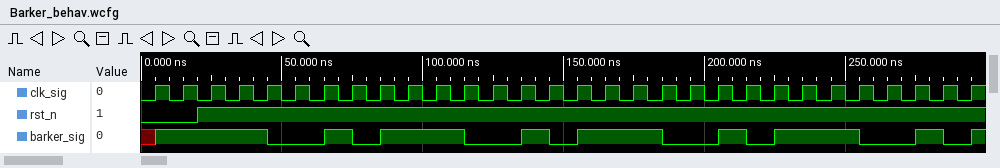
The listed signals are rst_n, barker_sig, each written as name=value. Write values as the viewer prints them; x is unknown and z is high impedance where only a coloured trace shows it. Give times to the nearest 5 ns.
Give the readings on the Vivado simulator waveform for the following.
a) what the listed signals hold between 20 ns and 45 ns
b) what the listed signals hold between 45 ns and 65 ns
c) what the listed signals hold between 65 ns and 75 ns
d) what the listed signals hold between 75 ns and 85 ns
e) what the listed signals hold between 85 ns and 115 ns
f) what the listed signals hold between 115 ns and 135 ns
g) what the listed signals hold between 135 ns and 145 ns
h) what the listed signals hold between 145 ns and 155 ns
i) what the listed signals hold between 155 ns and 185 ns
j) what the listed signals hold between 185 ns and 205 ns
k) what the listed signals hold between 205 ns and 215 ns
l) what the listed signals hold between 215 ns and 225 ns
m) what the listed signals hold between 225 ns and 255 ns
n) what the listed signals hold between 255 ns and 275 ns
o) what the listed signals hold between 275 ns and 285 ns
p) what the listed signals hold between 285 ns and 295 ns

rst_n=1, barker_sig=1
rst_n=1, barker_sig=0
rst_n=1, barker_sig=1
rst_n=1, barker_sig=0
rst_n=1, barker_sig=1
rst_n=1, barker_sig=0
rst_n=1, barker_sig=1
rst_n=1, barker_sig=0
rst_n=1, barker_sig=1
rst_n=1, barker_sig=0
rst_n=1, barker_sig=1
rst_n=1, barker_sig=0
rst_n=1, barker_sig=1
rst_n=1, barker_sig=0
rst_n=1, barker_sig=1
rst_n=1, barker_sig=0
